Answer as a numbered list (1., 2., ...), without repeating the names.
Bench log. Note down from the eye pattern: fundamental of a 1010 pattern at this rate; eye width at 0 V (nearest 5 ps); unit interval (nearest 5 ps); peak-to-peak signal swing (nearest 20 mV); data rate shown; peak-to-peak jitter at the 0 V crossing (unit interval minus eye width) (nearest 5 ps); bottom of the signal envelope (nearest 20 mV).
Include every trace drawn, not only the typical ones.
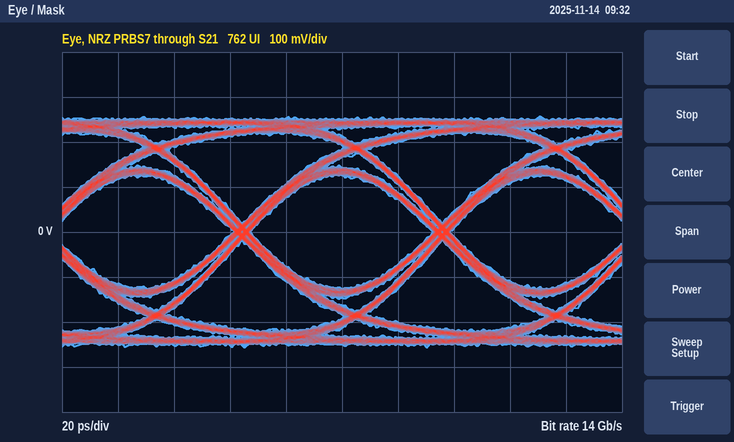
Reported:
1. 7 GHz
2. 65 ps
3. 70 ps
4. 520 mV
5. 14 Gb/s
6. 5 ps
7. -260 mV
